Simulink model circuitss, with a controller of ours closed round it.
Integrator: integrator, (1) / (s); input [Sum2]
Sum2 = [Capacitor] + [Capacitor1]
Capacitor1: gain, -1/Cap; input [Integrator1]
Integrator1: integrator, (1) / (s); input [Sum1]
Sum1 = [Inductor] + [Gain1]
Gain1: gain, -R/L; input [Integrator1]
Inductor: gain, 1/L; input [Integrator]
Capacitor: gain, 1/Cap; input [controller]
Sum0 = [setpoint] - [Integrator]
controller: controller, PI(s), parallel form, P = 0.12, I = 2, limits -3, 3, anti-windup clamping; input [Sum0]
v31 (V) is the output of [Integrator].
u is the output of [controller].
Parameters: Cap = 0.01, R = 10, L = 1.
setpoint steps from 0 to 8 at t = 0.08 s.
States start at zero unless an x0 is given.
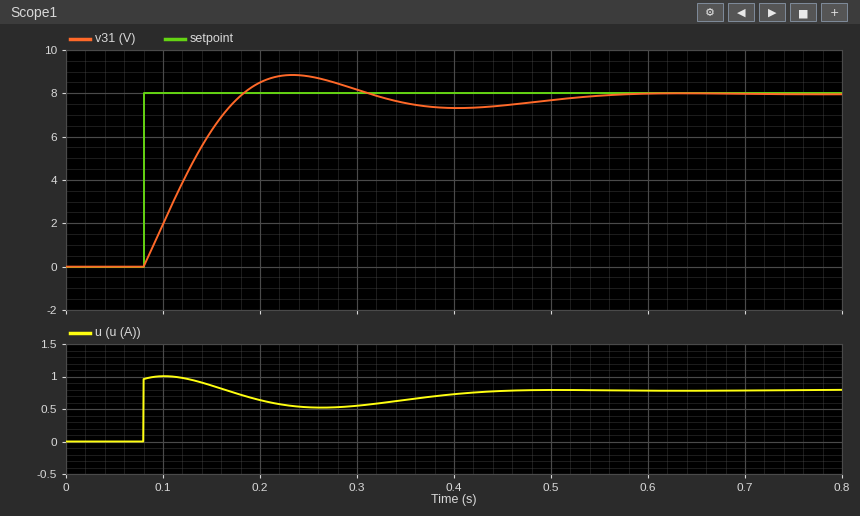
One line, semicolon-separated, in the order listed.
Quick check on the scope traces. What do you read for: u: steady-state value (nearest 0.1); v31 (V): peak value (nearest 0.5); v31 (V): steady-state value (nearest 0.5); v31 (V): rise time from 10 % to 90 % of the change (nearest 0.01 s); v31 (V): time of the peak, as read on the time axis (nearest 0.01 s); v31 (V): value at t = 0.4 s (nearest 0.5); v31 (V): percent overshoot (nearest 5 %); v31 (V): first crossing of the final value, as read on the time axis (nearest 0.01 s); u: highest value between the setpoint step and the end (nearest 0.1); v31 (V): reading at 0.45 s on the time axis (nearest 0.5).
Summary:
0.8; 9.0; 8.0; 0.08 s; 0.23 s; 7.5; 10 %; 0.18 s; 1.0; 7.5
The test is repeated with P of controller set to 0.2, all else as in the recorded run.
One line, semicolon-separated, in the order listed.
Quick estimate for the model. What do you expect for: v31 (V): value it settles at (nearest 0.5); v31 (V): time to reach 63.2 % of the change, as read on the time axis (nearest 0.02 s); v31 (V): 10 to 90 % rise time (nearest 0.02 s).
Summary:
8.0; 0.12 s; 0.06 s
